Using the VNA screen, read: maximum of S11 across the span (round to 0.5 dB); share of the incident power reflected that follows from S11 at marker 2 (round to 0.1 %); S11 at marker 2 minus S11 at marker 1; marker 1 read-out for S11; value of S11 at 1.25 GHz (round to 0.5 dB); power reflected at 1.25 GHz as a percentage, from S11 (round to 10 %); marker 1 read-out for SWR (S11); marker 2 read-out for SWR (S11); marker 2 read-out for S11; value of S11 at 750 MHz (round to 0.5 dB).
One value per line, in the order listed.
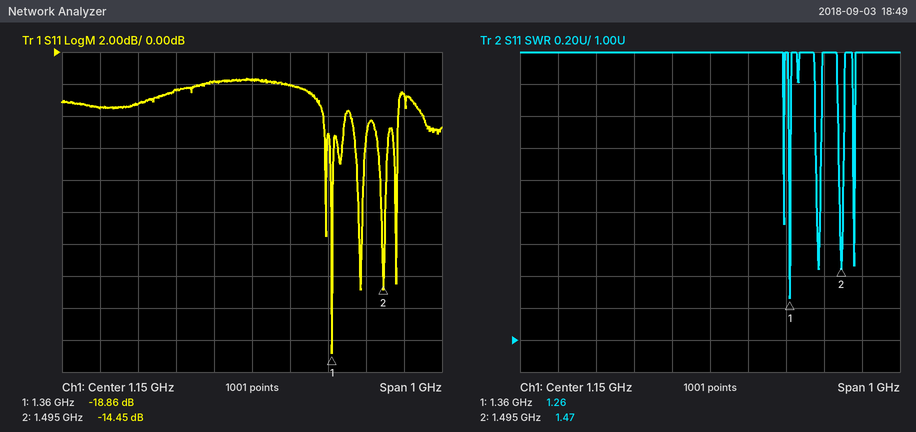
-1.5 dB
3.6 %
4.41 dB
-18.86 dB
-2.0 dB
60 %
1.26
1.47
-14.45 dB
-3.5 dB
